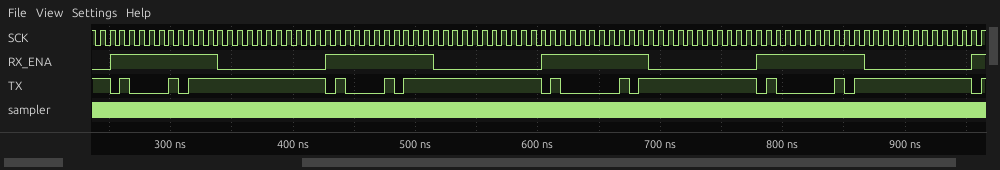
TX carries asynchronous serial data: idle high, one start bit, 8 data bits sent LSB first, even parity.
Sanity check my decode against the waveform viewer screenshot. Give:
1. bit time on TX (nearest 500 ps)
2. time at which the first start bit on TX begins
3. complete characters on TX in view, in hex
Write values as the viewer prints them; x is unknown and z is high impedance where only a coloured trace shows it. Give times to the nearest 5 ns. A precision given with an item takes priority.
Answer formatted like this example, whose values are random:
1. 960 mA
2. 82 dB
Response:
1. 8000 ps
2. 250 ns
3. A1, A1, 81, 81
